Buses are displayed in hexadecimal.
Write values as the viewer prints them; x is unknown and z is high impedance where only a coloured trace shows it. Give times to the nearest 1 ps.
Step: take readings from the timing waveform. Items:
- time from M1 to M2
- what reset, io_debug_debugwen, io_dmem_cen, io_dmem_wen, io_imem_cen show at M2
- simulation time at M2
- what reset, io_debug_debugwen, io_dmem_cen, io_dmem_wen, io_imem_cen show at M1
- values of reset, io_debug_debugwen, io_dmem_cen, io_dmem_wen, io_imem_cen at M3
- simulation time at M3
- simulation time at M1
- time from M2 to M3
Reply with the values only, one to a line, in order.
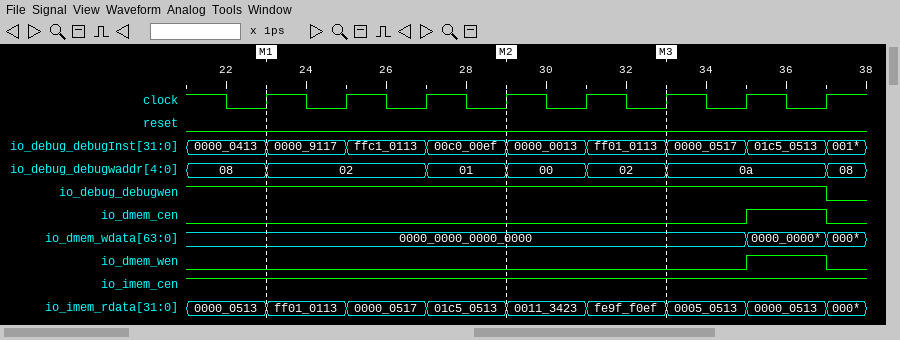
6 ps
reset=0, io_debug_debugwen=1, io_dmem_cen=0, io_dmem_wen=0, io_imem_cen=1
29 ps
reset=0, io_debug_debugwen=1, io_dmem_cen=0, io_dmem_wen=0, io_imem_cen=1
reset=0, io_debug_debugwen=1, io_dmem_cen=0, io_dmem_wen=0, io_imem_cen=1
33 ps
23 ps
4 ps
